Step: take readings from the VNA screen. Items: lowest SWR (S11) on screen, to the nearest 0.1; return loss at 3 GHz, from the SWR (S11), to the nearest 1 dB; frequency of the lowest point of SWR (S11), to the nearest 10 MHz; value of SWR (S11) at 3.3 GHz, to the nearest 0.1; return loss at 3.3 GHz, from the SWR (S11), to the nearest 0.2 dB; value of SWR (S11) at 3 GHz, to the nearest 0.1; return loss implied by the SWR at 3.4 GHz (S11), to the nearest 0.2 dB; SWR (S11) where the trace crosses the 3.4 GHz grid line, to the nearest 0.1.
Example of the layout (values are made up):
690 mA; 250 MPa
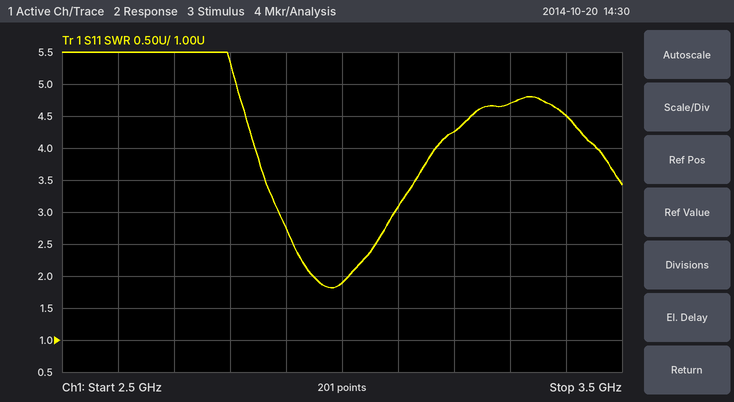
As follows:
1.8; 10 dB; 2.98 GHz; 4.7; 3.8 dB; 1.9; 4.0 dB; 4.5
